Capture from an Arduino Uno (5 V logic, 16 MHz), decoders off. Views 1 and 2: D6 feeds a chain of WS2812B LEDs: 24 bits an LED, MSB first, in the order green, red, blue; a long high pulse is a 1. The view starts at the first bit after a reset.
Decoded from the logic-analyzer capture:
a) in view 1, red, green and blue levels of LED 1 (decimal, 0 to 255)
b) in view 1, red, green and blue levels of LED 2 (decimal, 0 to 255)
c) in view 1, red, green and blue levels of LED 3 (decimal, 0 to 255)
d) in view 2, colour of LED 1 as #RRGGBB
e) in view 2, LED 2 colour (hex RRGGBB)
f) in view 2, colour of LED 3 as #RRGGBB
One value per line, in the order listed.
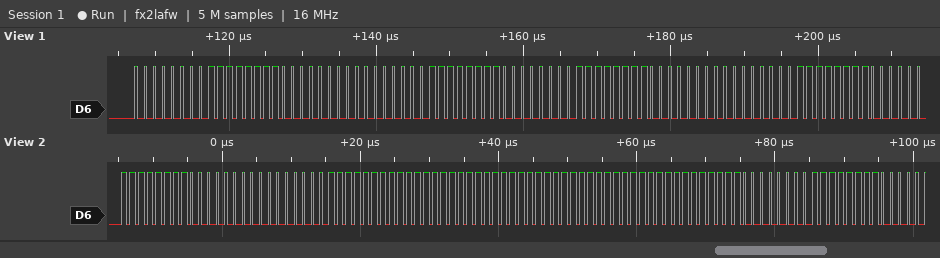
255, 0, 0
255, 0, 0
0, 255, 0
#00FF00
#FFFFFF
#FFFFFF
